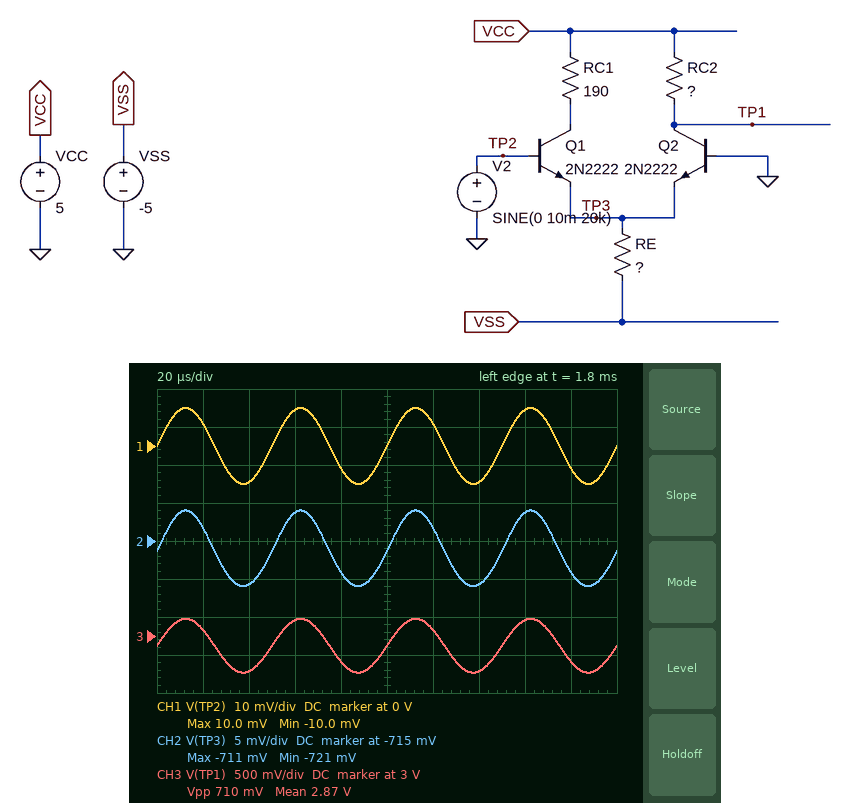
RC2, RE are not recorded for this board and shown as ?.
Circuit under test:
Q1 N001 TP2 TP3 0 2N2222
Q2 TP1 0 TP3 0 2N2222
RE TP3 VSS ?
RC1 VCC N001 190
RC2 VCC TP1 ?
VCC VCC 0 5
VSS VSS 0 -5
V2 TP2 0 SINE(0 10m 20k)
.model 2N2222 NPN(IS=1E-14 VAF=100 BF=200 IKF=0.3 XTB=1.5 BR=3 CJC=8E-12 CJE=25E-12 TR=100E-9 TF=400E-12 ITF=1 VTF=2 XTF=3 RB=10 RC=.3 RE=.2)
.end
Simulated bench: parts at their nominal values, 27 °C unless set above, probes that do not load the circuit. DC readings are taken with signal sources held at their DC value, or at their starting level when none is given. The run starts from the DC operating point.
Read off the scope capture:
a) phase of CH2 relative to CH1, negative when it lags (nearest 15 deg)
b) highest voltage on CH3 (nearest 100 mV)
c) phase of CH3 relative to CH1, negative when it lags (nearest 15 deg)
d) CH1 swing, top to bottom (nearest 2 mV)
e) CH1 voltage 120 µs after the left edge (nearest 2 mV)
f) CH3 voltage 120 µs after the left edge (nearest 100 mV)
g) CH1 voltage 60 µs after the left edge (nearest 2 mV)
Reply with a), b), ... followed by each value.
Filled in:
a) 0 deg
b) 3.2 V
c) 0 deg
d) 20 mV
e) 6 mV
f) 3.1 V
g) 10 mV
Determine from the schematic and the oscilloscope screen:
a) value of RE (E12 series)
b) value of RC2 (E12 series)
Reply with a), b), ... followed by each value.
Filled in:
a) 220 Ω
b) 220 Ω
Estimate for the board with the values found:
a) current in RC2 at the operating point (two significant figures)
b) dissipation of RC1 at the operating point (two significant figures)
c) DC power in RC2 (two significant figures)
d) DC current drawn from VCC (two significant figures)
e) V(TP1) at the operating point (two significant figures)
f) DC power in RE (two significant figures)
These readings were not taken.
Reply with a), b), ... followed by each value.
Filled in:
a) 9.7 mA
b) 18 mW
c) 21 mW
d) 19 mA
e) 2.9 V
f) 83 mW
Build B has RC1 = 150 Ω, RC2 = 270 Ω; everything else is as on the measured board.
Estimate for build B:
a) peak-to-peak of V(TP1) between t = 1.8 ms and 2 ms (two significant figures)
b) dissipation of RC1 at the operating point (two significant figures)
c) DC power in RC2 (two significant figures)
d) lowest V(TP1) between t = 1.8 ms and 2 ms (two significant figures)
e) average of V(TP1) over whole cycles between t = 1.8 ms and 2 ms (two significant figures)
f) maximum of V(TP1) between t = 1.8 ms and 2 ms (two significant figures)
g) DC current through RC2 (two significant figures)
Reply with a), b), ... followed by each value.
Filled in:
a) 870 mV
b) 14 mW
c) 25 mW
d) 2.0 V
e) 2.4 V
f) 2.8 V
g) 9.6 mA
